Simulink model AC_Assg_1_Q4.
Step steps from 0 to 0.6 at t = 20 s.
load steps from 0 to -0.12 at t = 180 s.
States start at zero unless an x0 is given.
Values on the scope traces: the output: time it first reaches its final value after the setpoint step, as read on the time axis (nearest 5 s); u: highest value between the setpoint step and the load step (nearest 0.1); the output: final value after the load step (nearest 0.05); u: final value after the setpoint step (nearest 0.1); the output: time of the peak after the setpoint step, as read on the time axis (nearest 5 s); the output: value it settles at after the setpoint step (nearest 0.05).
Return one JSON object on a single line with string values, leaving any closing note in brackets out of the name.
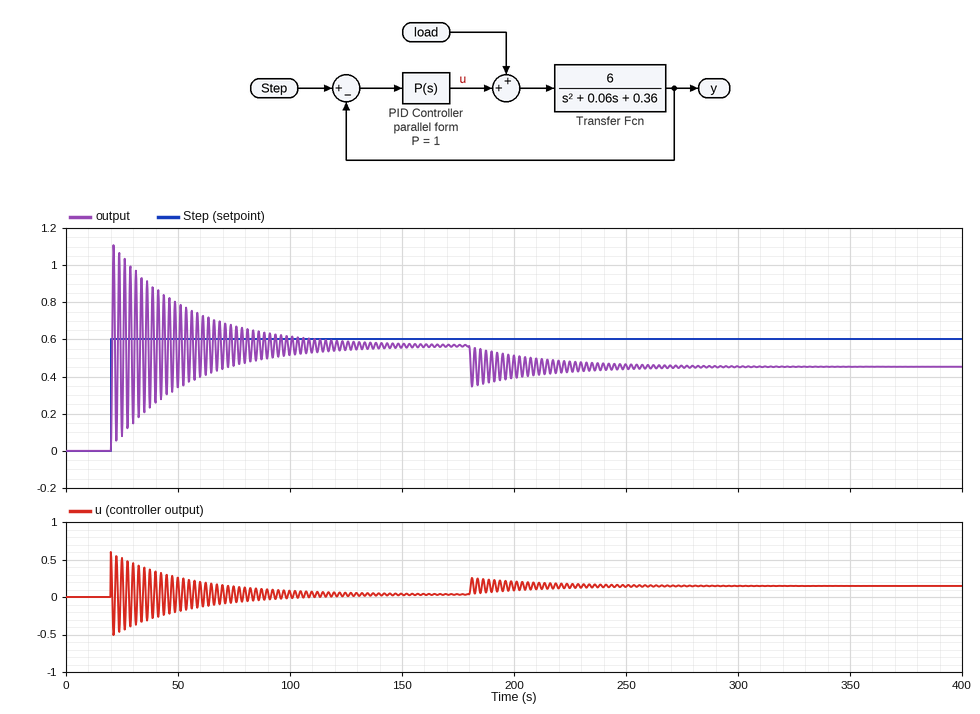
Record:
{"the output: time it first reaches its final value after the setpoint step, as read on the time axis": "20 s", "u: highest value between the setpoint step and the load step": "0.6", "the output: final value after the load step": "0.45", "u: final value after the setpoint step": "0.0", "the output: time of the peak after the setpoint step, as read on the time axis": "20 s", "the output: value it settles at after the setpoint step": "0.55"}
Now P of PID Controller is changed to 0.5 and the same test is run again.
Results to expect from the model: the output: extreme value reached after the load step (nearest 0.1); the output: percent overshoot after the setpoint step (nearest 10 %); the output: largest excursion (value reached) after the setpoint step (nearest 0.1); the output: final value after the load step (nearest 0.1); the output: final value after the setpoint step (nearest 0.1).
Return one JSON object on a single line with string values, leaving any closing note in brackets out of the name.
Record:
{"the output: extreme value reached after the load step": "0.1", "the output: percent overshoot after the setpoint step": "90 %", "the output: largest excursion (value reached) after the setpoint step": "1.0", "the output: final value after the load step": "0.3", "the output: final value after the setpoint step": "0.5"}
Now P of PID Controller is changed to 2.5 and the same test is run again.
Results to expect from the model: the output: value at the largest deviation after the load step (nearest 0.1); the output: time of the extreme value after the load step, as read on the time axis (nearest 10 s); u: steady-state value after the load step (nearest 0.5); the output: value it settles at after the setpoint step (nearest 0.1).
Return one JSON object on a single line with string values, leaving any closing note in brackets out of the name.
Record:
{"the output: value at the largest deviation after the load step": "0.5", "the output: time of the extreme value after the load step, as read on the time axis": "180 s", "u: steady-state value after the load step": "0.0", "the output: value it settles at after the setpoint step": "0.6"}
